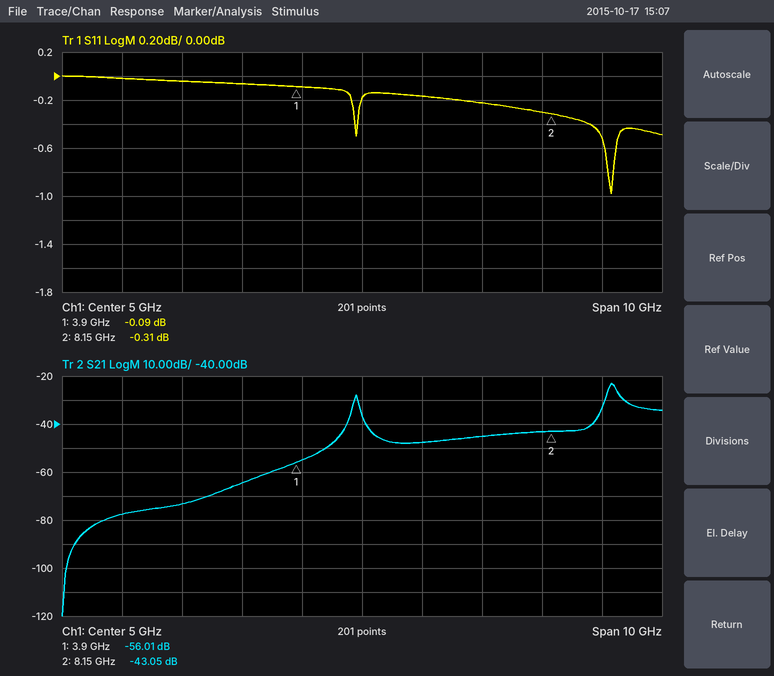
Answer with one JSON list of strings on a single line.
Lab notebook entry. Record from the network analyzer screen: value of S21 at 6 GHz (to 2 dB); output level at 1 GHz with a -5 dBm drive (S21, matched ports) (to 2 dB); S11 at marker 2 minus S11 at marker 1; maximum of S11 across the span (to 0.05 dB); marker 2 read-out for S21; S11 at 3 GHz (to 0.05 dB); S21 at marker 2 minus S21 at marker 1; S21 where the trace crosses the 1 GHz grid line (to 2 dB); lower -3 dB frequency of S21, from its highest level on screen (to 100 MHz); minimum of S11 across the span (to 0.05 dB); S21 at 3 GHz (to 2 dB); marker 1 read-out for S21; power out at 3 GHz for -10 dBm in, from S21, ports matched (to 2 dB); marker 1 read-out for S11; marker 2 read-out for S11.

["-48 dB", "-82 dBm", "-0.22 dB", "0.00 dB", "-43.05 dB", "-0.05 dB", "12.96 dB", "-78 dB", "9.1 GHz", "-1.00 dB", "-64 dB", "-56.01 dB", "-74 dBm", "-0.09 dB", "-0.31 dB"]
